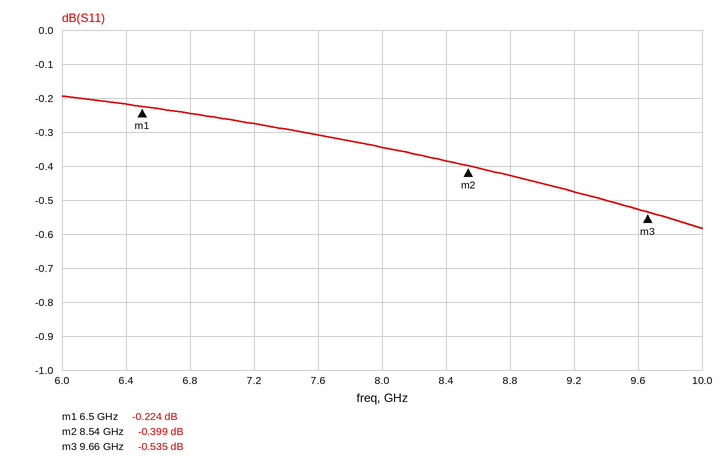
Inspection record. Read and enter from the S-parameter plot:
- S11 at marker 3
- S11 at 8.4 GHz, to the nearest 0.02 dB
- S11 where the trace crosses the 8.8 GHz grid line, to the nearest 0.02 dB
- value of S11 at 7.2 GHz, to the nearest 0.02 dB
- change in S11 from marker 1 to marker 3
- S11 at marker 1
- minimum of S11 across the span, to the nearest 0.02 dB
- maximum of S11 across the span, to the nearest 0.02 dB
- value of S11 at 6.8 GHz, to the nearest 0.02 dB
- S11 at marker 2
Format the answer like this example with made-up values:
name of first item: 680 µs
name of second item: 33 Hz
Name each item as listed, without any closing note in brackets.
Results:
S11 at marker 3: -0.535 dB
S11 at 8.4 GHz, to the nearest 0.02 dB: -0.38 dB
S11 where the trace crosses the 8.8 GHz grid line, to the nearest 0.02 dB: -0.42 dB
value of S11 at 7.2 GHz, to the nearest 0.02 dB: -0.28 dB
change in S11 from marker 1 to marker 3: -0.311 dB
S11 at marker 1: -0.224 dB
minimum of S11 across the span, to the nearest 0.02 dB: -0.58 dB
maximum of S11 across the span, to the nearest 0.02 dB: -0.20 dB
value of S11 at 6.8 GHz, to the nearest 0.02 dB: -0.24 dB
S11 at marker 2: -0.399 dB
